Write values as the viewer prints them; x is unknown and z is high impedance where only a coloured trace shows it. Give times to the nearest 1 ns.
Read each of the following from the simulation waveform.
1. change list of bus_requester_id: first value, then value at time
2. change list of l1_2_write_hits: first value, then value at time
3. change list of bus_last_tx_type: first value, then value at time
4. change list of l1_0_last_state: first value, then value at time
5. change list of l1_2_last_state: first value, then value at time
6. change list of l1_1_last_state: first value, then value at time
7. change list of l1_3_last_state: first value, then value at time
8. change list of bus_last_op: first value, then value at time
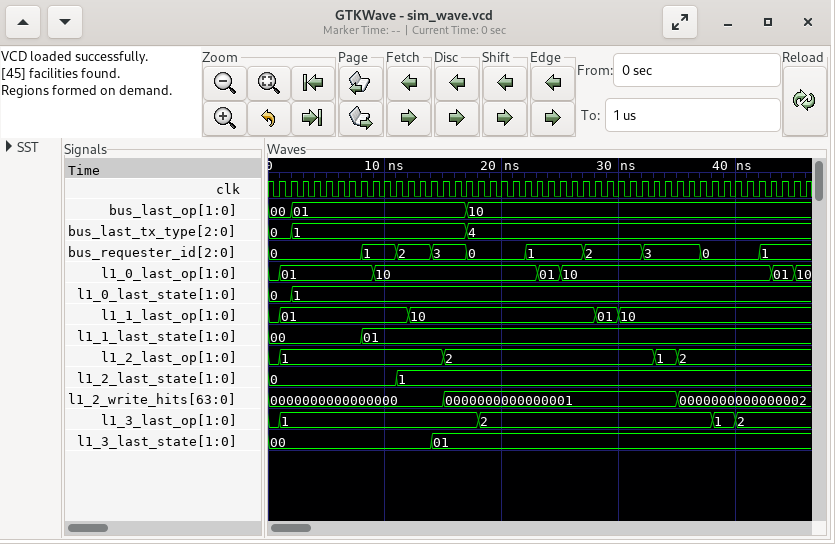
0, 1 at 8 ns, 2 at 11 ns, 3 at 14 ns, 0 at 17 ns, 1 at 22 ns, 2 at 27 ns, 3 at 32 ns, 0 at 37 ns, 1 at 42 ns
0000000000000000, 0000000000000001 at 15 ns, 0000000000000002 at 35 ns
0, 1 at 2 ns, 4 at 17 ns
0, 1 at 2 ns
0, 1 at 11 ns
00, 01 at 8 ns
00, 01 at 14 ns
00, 01 at 2 ns, 10 at 17 ns
